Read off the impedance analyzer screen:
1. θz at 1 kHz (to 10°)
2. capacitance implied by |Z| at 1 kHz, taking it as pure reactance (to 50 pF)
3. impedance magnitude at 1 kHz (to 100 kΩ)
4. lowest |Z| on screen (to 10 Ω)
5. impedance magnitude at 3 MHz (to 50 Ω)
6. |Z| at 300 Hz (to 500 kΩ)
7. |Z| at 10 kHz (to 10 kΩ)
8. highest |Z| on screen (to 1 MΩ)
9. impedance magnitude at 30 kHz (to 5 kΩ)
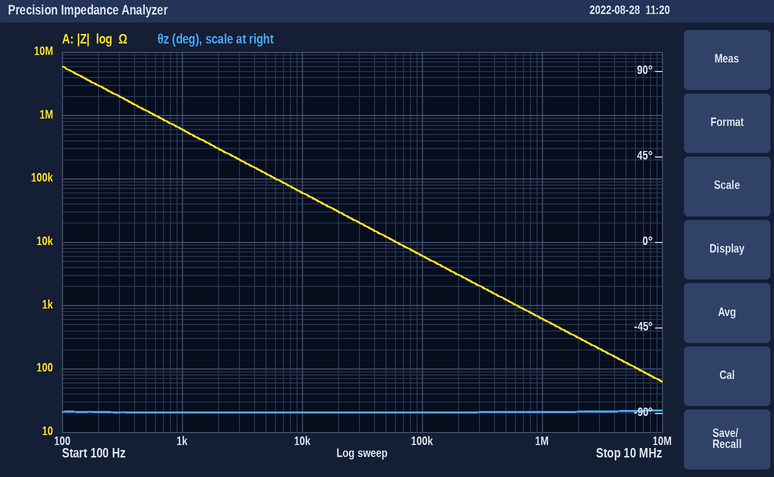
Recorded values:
-90°
250 pF
600 kΩ
60 Ω
200 Ω
2.0 MΩ
60 kΩ
6 MΩ
20 kΩ
